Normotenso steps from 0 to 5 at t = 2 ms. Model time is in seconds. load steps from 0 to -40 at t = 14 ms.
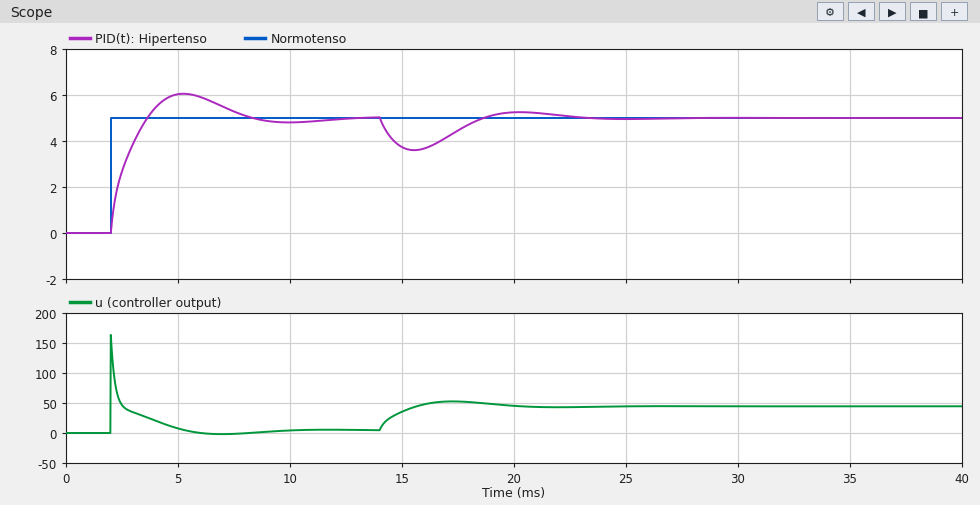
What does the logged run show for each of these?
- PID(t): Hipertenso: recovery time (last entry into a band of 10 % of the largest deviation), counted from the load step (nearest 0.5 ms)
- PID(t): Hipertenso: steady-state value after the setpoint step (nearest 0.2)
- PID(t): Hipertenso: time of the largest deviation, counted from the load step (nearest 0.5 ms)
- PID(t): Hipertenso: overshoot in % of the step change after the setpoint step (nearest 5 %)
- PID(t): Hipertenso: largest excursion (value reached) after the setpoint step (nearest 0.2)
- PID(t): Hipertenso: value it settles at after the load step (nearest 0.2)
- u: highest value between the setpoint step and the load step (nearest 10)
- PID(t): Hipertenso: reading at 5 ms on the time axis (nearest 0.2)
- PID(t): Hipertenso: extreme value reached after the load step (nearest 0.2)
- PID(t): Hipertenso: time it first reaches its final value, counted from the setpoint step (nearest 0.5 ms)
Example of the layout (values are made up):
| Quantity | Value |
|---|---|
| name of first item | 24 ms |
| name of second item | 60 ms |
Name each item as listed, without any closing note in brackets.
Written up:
| Quantity | Value |
|---|---|
| PID(t): Hipertenso: recovery time (last entry into a band of 10 % of the largest deviation), counted from the load step | 8.0 ms |
| PID(t): Hipertenso: steady-state value after the setpoint step | 5.0 |
| PID(t): Hipertenso: time of the largest deviation, counted from the load step | 1.5 ms |
| PID(t): Hipertenso: overshoot in % of the step change after the setpoint step | 20 % |
| PID(t): Hipertenso: largest excursion (value reached) after the setpoint step | 6.0 |
| PID(t): Hipertenso: value it settles at after the load step | 5.0 |
| u: highest value between the setpoint step and the load step | 160 |
| PID(t): Hipertenso: reading at 5 ms on the time axis | 6.0 |
| PID(t): Hipertenso: extreme value reached after the load step | 3.6 |
| PID(t): Hipertenso: time it first reaches its final value, counted from the setpoint step | 1.5 ms |
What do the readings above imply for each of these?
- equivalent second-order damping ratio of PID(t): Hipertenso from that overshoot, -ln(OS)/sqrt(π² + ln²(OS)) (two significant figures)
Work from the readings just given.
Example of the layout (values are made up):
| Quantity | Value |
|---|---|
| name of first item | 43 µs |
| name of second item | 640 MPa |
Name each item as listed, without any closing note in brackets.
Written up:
| Quantity | Value |
|---|---|
| equivalent second-order damping ratio of PID(t): Hipertenso from that overshoot, -ln(OS)/sqrt(π² + ln²(OS)) | 0.46 |
